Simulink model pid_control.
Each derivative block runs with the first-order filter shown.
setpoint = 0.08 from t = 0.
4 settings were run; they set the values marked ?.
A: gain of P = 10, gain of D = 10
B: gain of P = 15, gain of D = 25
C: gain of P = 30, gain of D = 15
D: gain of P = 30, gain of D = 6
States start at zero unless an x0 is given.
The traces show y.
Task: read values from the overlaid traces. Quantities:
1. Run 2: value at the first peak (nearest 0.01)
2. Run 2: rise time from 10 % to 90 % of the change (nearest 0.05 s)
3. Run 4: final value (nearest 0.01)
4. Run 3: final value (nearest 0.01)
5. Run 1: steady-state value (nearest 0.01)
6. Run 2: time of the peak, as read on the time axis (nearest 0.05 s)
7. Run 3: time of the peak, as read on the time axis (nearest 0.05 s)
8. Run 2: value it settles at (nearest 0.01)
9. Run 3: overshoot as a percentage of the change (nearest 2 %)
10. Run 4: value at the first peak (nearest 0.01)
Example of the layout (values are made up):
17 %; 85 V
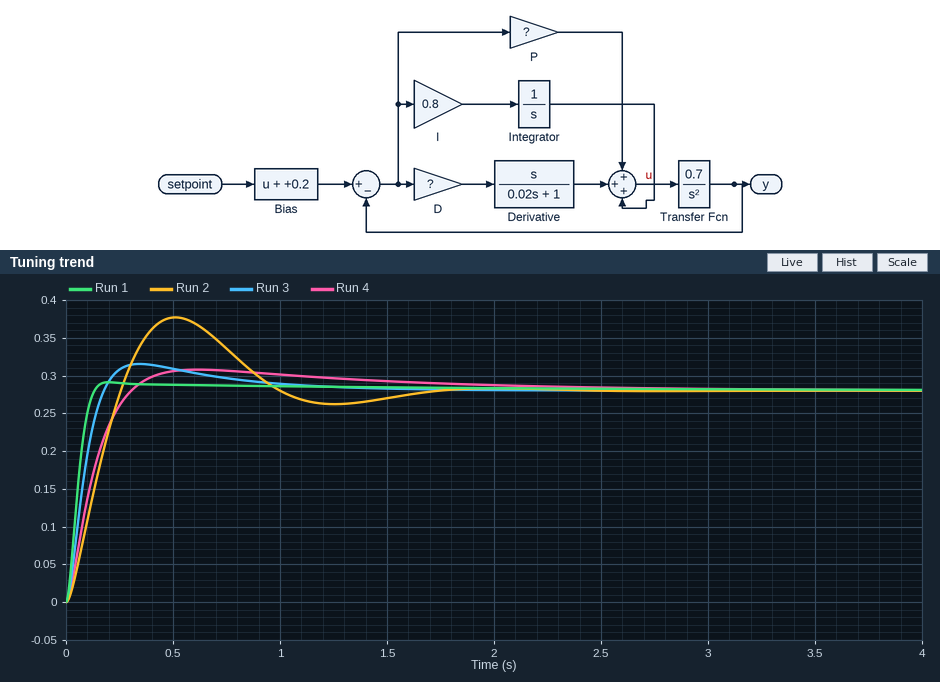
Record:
0.38; 0.20 s; 0.28; 0.28; 0.28; 0.50 s; 0.35 s; 0.28; 12 %; 0.31
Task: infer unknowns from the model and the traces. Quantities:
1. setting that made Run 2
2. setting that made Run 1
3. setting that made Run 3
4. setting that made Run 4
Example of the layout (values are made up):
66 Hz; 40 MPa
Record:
D; B; C; A
